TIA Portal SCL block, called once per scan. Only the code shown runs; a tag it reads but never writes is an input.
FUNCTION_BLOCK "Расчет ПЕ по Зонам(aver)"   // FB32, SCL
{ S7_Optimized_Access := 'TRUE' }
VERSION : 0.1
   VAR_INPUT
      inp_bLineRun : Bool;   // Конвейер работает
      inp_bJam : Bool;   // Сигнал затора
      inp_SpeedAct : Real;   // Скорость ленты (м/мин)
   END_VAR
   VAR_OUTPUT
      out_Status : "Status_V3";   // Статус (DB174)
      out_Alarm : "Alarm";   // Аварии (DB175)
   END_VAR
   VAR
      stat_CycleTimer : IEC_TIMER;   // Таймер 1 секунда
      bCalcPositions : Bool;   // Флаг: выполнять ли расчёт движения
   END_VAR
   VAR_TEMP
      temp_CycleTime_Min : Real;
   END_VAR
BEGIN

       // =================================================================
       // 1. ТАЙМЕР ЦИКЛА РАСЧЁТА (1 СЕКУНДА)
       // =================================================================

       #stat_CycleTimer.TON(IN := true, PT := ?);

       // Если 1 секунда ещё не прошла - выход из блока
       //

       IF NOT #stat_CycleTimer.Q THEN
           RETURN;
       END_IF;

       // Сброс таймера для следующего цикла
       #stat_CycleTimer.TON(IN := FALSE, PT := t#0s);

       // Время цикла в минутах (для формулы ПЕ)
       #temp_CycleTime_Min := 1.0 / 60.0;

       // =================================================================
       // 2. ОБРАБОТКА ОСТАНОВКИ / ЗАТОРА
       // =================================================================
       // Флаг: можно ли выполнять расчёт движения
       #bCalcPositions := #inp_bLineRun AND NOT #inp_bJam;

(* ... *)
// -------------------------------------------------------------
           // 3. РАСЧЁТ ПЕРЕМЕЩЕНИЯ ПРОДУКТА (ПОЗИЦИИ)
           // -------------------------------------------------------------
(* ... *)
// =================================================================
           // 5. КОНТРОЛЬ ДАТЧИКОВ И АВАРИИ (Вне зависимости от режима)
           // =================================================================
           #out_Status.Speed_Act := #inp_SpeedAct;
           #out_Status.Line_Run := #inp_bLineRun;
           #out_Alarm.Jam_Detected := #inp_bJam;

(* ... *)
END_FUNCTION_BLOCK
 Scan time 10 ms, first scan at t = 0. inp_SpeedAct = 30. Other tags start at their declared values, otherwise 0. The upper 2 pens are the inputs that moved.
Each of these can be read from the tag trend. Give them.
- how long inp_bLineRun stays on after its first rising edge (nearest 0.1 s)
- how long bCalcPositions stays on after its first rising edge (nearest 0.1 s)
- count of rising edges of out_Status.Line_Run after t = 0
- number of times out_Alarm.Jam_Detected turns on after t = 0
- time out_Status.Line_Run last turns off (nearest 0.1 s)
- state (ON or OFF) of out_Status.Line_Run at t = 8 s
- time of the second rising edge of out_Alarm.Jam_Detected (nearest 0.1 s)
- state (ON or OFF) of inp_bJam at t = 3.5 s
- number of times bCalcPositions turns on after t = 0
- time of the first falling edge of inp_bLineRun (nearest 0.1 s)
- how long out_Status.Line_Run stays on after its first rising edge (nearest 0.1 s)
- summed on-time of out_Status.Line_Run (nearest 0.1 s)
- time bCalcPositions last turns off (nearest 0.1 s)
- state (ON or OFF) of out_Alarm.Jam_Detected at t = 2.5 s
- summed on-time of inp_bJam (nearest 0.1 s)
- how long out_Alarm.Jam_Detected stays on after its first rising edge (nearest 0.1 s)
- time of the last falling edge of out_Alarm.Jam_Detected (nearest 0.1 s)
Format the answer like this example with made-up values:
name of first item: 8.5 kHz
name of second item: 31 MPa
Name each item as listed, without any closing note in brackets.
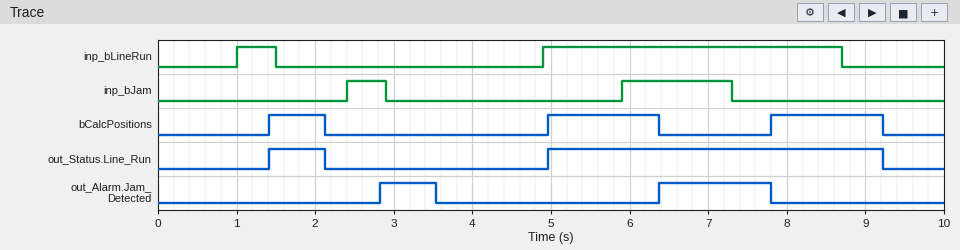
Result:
how long inp_bLineRun stays on after its first rising edge: 0.5 s
how long bCalcPositions stays on after its first rising edge: 0.7 s
count of rising edges of out_Status.Line_Run after t = 0: 2
number of times out_Alarm.Jam_Detected turns on after t = 0: 2
time out_Status.Line_Run last turns off: 9.2 s
state (ON or OFF) of out_Status.Line_Run at t = 8 s: ON
time of the second rising edge of out_Alarm.Jam_Detected: 6.4 s
state (ON or OFF) of inp_bJam at t = 3.5 s: OFF
number of times bCalcPositions turns on after t = 0: 3
time of the first falling edge of inp_bLineRun: 1.5 s
how long out_Status.Line_Run stays on after its first rising edge: 0.7 s
summed on-time of out_Status.Line_Run: 5.0 s
time bCalcPositions last turns off: 9.2 s
state (ON or OFF) of out_Alarm.Jam_Detected at t = 2.5 s: OFF
summed on-time of inp_bJam: 1.9 s
how long out_Alarm.Jam_Detected stays on after its first rising edge: 0.7 s
time of the last falling edge of out_Alarm.Jam_Detected: 7.8 s
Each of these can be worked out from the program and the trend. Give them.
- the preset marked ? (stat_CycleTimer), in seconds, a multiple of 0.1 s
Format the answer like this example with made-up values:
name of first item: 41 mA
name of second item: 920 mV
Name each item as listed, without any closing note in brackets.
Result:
the preset marked ? (stat_CycleTimer), in seconds, a multiple of 0.1 s: 0.7 s
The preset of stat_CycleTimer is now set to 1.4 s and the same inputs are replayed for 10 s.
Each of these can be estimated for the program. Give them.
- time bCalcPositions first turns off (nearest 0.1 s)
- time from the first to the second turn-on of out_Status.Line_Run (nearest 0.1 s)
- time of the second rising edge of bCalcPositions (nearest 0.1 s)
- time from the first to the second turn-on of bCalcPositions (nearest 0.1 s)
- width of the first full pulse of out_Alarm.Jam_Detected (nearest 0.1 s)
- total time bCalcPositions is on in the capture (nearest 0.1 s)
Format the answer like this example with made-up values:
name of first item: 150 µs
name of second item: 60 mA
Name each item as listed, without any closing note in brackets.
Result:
time bCalcPositions first turns off: 2.8 s
time from the first to the second turn-on of out_Status.Line_Run: 4.2 s
time of the second rising edge of bCalcPositions: 5.6 s
time from the first to the second turn-on of bCalcPositions: 4.2 s
width of the first full pulse of out_Alarm.Jam_Detected: 1.4 s
total time bCalcPositions is on in the capture: 4.2 s
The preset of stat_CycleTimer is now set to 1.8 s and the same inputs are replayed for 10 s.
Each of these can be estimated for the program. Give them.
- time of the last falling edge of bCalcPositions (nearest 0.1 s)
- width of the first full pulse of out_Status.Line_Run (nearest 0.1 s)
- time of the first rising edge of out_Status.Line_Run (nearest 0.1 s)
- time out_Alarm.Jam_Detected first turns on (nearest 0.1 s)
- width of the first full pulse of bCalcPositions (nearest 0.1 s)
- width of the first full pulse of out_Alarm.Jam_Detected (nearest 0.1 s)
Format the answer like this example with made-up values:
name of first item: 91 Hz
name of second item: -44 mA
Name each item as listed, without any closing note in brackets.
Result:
time of the last falling edge of bCalcPositions: 7.2 s
width of the first full pulse of out_Status.Line_Run: 3.6 s
time of the first rising edge of out_Status.Line_Run: 5.4 s
time out_Alarm.Jam_Detected first turns on: 7.2 s
width of the first full pulse of bCalcPositions: 1.8 s
width of the first full pulse of out_Alarm.Jam_Detected: 1.8 s
